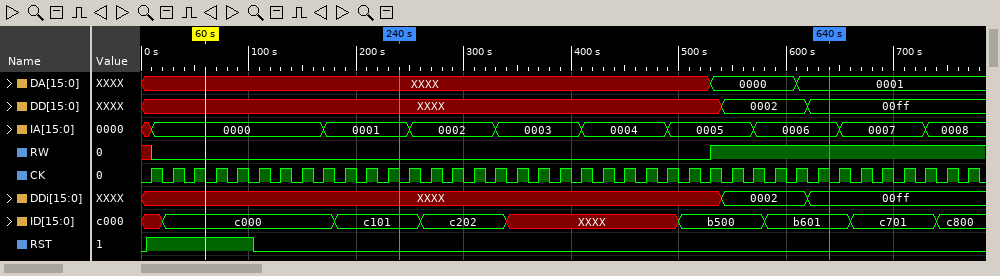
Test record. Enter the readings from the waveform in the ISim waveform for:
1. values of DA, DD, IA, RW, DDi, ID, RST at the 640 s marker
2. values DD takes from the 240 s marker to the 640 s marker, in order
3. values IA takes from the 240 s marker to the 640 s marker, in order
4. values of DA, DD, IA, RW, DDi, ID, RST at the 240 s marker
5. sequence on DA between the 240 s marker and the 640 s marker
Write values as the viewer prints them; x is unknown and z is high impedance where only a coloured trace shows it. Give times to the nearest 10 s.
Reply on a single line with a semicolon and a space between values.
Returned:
DA=0001, DD=00ff, IA=0006, RW=1, DDi=00ff, ID=b601, RST=0; XXXX, 0002, 00ff; 0001, 0002, 0003, 0004, 0005, 0006; DA=XXXX, DD=XXXX, IA=0001, RW=0, DDi=XXXX, ID=c101, RST=0; XXXX, 0000, 0001
